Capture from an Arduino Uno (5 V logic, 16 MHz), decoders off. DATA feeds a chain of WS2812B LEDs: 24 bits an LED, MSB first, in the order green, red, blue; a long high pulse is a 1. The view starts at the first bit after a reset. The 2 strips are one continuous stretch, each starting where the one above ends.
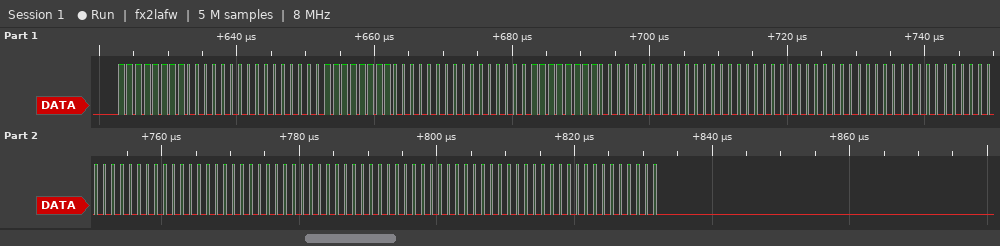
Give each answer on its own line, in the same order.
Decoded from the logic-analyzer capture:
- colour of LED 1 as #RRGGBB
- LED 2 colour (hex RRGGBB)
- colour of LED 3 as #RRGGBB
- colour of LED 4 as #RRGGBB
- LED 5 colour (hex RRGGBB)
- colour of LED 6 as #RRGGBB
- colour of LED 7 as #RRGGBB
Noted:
#00FF00
#00FF00
#00FF00
#000000
#000000
#000000
#000000
